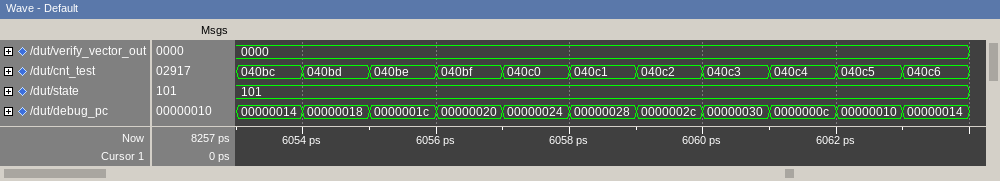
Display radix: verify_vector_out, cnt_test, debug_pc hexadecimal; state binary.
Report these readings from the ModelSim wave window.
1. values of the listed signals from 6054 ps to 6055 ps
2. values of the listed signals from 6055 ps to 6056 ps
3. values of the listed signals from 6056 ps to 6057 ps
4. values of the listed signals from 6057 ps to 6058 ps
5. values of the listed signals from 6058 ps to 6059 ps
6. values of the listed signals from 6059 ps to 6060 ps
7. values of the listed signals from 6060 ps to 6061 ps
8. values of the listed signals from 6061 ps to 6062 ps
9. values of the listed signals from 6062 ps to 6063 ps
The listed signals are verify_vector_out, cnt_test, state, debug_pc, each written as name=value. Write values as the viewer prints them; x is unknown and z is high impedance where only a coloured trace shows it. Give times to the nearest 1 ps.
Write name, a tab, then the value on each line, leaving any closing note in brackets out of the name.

values of the listed signals from 6054 ps to 6055 ps	verify_vector_out=0000, cnt_test=040bd, state=101, debug_pc=00000018
values of the listed signals from 6055 ps to 6056 ps	verify_vector_out=0000, cnt_test=040be, state=101, debug_pc=0000001c
values of the listed signals from 6056 ps to 6057 ps	verify_vector_out=0000, cnt_test=040bf, state=101, debug_pc=00000020
values of the listed signals from 6057 ps to 6058 ps	verify_vector_out=0000, cnt_test=040c0, state=101, debug_pc=00000024
values of the listed signals from 6058 ps to 6059 ps	verify_vector_out=0000, cnt_test=040c1, state=101, debug_pc=00000028
values of the listed signals from 6059 ps to 6060 ps	verify_vector_out=0000, cnt_test=040c2, state=101, debug_pc=0000002c
values of the listed signals from 6060 ps to 6061 ps	verify_vector_out=0000, cnt_test=040c3, state=101, debug_pc=00000030
values of the listed signals from 6061 ps to 6062 ps	verify_vector_out=0000, cnt_test=040c4, state=101, debug_pc=0000000c
values of the listed signals from 6062 ps to 6063 ps	verify_vector_out=0000, cnt_test=040c5, state=101, debug_pc=00000010
